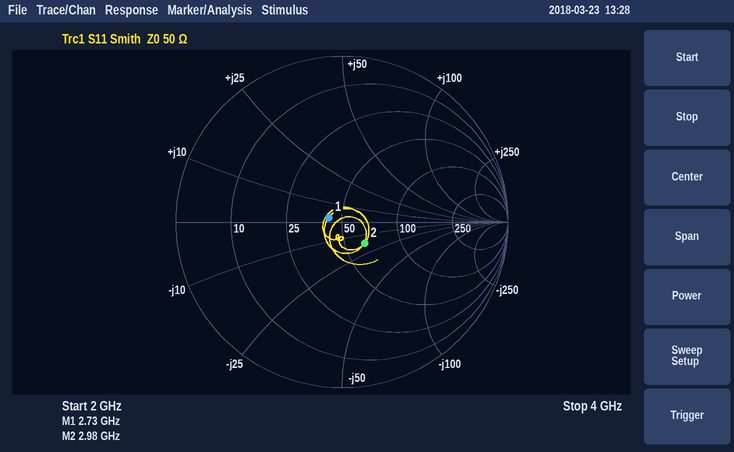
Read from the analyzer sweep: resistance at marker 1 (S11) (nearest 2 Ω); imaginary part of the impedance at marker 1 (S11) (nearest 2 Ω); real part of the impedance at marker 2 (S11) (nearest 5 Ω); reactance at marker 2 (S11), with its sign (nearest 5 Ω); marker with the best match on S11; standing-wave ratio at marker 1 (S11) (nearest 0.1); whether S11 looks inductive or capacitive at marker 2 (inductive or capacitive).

42 Ω
+2 Ω
65 Ω
-15 Ω
marker 1
1.2
capacitive
